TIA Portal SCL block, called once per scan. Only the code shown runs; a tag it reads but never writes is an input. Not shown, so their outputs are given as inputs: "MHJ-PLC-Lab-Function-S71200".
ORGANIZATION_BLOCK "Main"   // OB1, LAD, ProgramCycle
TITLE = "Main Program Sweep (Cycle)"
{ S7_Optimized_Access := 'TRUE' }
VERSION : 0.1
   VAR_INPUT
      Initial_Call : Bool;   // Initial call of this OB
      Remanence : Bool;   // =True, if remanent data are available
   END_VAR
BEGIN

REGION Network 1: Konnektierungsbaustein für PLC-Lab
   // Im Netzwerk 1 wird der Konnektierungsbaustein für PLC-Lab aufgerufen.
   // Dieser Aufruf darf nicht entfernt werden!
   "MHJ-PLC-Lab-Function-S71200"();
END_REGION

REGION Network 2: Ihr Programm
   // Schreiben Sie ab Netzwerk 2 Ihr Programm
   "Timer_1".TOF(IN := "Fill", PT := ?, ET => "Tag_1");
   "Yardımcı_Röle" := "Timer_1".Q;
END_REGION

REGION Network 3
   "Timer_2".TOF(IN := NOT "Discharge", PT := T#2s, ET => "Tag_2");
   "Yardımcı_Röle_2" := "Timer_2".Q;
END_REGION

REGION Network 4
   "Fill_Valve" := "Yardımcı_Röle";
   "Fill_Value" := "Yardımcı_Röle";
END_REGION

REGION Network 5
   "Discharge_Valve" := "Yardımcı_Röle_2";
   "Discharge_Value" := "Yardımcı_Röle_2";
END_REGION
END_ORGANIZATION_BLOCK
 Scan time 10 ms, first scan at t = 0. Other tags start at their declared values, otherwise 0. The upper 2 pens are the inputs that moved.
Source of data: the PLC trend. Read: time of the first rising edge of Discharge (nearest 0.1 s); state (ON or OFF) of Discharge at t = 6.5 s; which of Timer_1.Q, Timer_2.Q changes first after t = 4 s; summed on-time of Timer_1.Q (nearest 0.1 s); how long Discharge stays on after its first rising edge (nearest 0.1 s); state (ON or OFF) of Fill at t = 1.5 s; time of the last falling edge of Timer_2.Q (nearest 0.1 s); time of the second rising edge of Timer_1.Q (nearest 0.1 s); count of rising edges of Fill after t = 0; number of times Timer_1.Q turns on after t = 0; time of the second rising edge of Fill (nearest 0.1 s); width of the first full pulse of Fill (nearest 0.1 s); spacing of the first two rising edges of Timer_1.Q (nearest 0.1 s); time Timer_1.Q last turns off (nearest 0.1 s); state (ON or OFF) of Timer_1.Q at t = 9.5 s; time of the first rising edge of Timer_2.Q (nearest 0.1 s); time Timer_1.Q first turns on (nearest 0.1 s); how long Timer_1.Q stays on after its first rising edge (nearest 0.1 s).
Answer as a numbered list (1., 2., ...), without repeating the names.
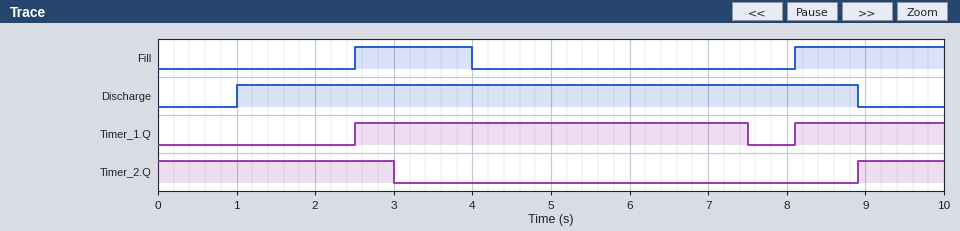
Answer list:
1. 1.0 s
2. ON
3. Timer_1.Q
4. 6.9 s
5. 7.9 s
6. OFF
7. 3.0 s
8. 8.1 s
9. 2
10. 2
11. 8.1 s
12. 1.5 s
13. 5.6 s
14. 7.5 s
15. ON
16. 8.9 s
17. 2.5 s
18. 5.0 s
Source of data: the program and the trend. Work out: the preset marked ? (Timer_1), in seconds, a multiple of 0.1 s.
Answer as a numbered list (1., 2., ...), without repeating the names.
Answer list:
1. 3.5 s
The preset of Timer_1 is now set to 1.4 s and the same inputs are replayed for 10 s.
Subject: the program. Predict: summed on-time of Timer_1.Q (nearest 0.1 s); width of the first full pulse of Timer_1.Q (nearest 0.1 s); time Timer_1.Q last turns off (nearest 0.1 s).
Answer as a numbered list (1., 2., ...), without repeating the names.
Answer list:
1. 4.8 s
2. 2.9 s
3. 5.4 s
